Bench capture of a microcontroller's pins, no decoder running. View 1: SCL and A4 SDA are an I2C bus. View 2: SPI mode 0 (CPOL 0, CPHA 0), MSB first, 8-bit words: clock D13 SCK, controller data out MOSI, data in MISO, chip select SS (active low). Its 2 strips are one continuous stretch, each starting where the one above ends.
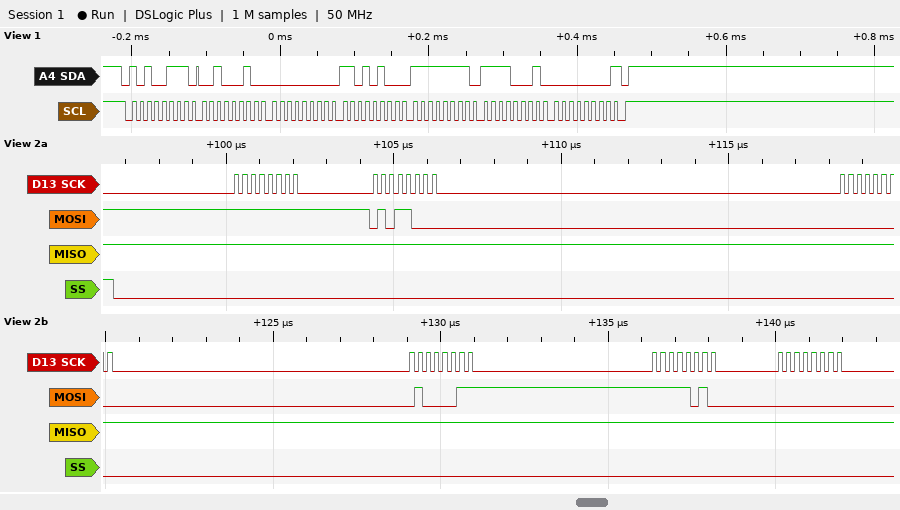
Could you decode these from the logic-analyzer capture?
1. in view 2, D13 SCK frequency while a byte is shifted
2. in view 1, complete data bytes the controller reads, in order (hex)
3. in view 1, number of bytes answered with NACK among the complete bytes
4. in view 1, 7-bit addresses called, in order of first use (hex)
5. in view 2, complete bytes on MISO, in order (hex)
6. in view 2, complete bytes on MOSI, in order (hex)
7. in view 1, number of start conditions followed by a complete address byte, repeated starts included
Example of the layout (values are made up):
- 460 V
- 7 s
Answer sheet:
- 4 MHz
- 22 00 D4 FF F1 00
- 1
- 0x53
- FF FF FF FF FF FF
- FF 58 00 43 FA 00
- 1
